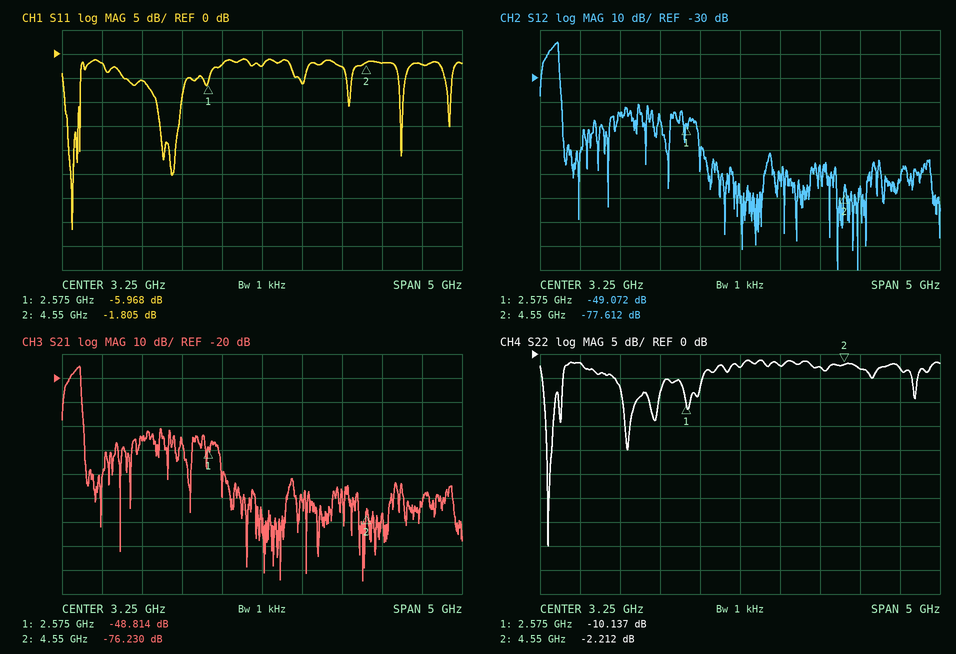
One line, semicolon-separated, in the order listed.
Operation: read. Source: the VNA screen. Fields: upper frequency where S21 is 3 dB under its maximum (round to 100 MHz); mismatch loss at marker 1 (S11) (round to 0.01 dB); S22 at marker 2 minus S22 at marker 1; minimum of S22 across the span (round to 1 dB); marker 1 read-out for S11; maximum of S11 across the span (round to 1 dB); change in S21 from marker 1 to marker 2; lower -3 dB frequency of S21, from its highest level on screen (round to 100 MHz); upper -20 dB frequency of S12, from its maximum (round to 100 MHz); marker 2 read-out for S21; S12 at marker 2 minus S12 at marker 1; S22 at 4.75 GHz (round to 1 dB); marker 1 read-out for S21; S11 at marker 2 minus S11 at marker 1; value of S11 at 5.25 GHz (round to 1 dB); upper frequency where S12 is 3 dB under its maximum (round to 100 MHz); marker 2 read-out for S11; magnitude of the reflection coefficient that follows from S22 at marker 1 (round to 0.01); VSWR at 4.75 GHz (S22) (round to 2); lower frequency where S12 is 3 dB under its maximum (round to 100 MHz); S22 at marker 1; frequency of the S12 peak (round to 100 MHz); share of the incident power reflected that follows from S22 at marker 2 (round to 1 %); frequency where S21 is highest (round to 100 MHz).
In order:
1.0 GHz; 1.27 dB; 7.925 dB; -40 dB; -5.968 dB; -1 dB; -27.416 dB; 900 MHz; 1.0 GHz; -76.230 dB; -28.540 dB; -3 dB; -48.814 dB; 4.163 dB; -2 dB; 1.0 GHz; -1.805 dB; 0.31; 6; 900 MHz; -10.137 dB; 1.0 GHz; 60 %; 1.0 GHz
